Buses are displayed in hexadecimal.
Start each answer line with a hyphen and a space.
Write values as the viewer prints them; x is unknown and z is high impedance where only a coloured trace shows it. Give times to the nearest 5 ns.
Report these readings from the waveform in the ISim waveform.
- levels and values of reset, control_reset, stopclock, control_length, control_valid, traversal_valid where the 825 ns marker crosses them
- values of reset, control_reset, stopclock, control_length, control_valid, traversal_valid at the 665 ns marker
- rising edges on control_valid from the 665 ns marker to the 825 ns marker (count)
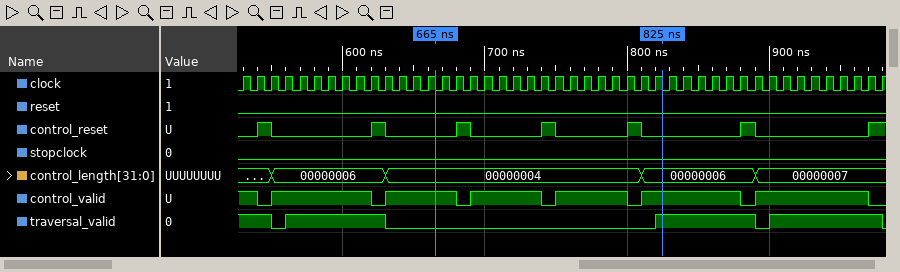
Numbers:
- reset=0, control_reset=0, stopclock=0, control_length=00000006, control_valid=1, traversal_valid=1
- reset=0, control_reset=0, stopclock=0, control_length=00000004, control_valid=1, traversal_valid=0
- 3
